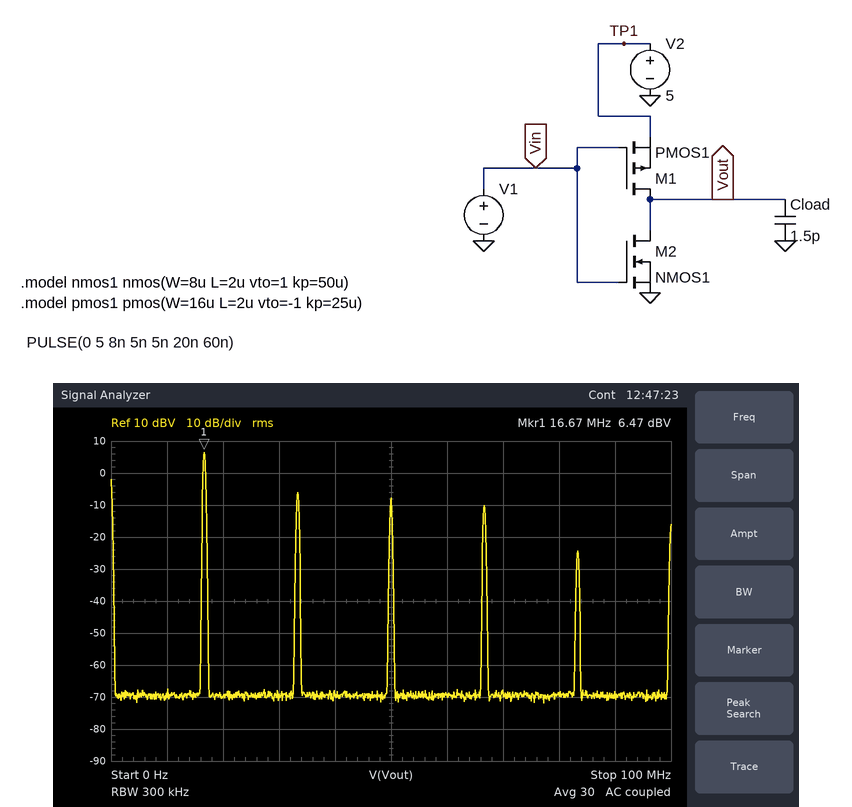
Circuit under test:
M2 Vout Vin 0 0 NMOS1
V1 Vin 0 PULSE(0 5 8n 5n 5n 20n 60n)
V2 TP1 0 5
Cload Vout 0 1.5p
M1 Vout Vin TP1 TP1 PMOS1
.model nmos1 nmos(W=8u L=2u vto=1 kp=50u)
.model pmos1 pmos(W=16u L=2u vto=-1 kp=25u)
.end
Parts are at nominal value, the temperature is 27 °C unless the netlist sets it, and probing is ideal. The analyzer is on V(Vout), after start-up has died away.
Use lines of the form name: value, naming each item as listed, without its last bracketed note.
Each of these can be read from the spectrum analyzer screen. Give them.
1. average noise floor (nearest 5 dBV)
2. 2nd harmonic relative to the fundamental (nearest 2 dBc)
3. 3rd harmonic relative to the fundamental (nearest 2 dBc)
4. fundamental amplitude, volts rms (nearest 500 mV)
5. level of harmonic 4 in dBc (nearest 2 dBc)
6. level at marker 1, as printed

average noise floor: -70 dBV
2nd harmonic relative to the fundamental: -12 dBc
3rd harmonic relative to the fundamental: -14 dBc
fundamental amplitude, volts rms: 2.0 V
level of harmonic 4 in dBc: -16 dBc
level at marker 1, as printed: 6.47 dBV
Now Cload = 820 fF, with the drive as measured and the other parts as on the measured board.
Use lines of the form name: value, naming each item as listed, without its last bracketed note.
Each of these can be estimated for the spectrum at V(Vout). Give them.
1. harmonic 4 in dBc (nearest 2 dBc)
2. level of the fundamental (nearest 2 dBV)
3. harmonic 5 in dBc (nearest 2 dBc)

harmonic 4 in dBc: -14 dBc
level of the fundamental: 6 dBV
harmonic 5 in dBc: -28 dBc
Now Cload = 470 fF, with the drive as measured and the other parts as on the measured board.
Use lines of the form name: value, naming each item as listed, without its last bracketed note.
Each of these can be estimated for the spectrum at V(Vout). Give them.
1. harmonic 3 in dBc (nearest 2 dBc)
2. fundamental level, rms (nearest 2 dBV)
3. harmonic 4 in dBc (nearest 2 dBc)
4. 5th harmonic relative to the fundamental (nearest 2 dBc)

harmonic 3 in dBc: -12 dBc
fundamental level, rms: 6 dBV
harmonic 4 in dBc: -14 dBc
5th harmonic relative to the fundamental: -26 dBc
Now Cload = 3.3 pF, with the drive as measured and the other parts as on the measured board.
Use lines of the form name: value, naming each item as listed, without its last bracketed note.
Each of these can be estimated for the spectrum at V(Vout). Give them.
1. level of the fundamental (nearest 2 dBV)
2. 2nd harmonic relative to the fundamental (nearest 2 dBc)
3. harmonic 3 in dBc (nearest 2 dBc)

level of the fundamental: 6 dBV
2nd harmonic relative to the fundamental: -14 dBc
harmonic 3 in dBc: -18 dBc
